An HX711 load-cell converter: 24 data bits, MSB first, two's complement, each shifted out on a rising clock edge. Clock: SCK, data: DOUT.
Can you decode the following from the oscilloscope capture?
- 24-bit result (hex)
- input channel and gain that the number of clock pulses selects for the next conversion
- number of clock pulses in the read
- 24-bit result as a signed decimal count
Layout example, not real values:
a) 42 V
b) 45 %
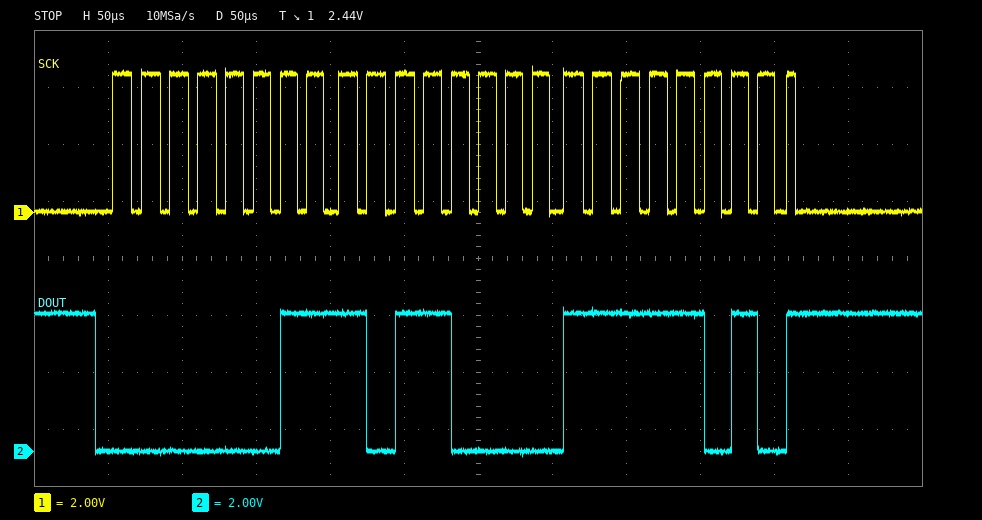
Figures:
a) 0x03B0FA
b) channel A, gain 128
c) 25
d) 241914
